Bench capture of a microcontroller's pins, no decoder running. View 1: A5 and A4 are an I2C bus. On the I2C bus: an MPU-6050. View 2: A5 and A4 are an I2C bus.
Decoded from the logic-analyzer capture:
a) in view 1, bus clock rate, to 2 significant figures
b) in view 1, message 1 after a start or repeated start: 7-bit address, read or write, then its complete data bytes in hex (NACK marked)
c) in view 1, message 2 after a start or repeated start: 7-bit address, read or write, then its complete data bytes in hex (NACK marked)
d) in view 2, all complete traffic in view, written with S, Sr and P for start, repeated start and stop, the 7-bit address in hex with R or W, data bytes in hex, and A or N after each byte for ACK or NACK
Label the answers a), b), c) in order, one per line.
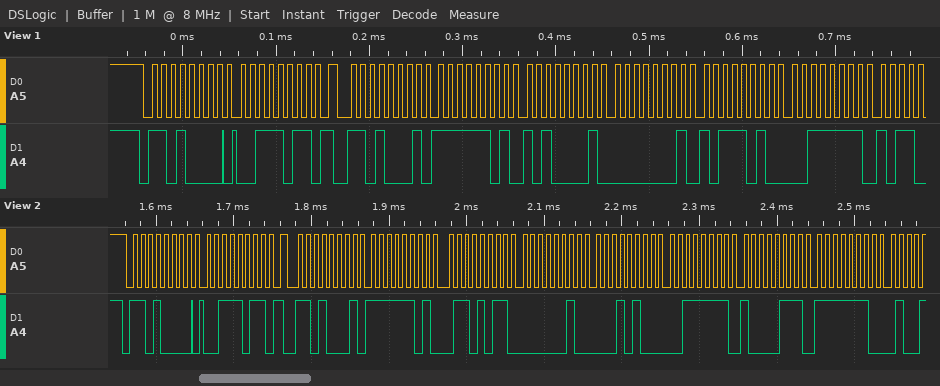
a) 100 kHz
b) 0x68 write: 3B
c) 0x68 read: FD A1 01 BA 3F
d) S 68W A 3B A Sr 68R A FD A 6B A 02 A 14 A 3F A 87 A FE A
